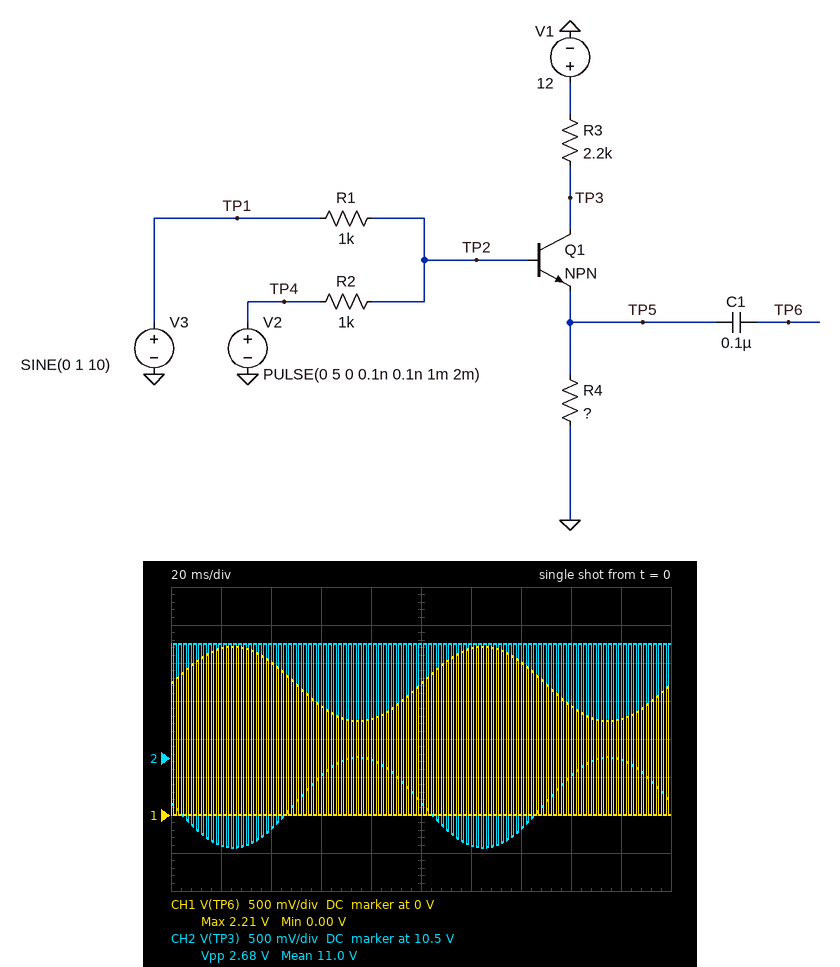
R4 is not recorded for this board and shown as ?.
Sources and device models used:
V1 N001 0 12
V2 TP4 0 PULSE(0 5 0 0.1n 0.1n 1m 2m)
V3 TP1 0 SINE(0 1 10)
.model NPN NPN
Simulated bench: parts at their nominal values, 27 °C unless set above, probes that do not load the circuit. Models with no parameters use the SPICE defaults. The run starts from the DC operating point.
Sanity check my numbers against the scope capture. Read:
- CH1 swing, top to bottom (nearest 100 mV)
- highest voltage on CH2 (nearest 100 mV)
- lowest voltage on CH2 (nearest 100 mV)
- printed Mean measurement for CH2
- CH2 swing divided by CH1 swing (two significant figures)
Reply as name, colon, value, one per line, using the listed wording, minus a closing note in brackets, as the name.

CH1 swing, top to bottom: 2.2 V
highest voltage on CH2: 12.0 V
lowest voltage on CH2: 9.3 V
printed Mean measurement for CH2: 11.0 V
CH2 swing divided by CH1 swing: 1.2
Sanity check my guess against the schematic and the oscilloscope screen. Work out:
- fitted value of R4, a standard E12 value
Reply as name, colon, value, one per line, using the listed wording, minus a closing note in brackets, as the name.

fitted value of R4, a standard E12 value: 1.8 kΩ
